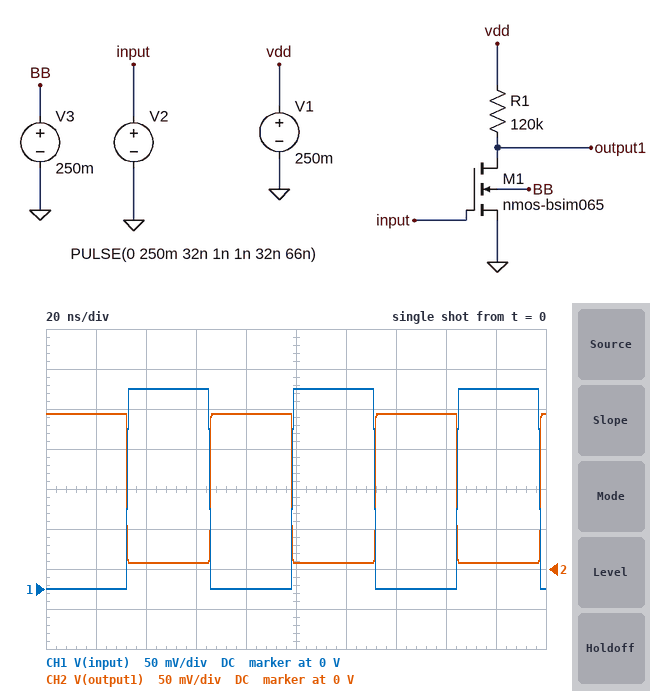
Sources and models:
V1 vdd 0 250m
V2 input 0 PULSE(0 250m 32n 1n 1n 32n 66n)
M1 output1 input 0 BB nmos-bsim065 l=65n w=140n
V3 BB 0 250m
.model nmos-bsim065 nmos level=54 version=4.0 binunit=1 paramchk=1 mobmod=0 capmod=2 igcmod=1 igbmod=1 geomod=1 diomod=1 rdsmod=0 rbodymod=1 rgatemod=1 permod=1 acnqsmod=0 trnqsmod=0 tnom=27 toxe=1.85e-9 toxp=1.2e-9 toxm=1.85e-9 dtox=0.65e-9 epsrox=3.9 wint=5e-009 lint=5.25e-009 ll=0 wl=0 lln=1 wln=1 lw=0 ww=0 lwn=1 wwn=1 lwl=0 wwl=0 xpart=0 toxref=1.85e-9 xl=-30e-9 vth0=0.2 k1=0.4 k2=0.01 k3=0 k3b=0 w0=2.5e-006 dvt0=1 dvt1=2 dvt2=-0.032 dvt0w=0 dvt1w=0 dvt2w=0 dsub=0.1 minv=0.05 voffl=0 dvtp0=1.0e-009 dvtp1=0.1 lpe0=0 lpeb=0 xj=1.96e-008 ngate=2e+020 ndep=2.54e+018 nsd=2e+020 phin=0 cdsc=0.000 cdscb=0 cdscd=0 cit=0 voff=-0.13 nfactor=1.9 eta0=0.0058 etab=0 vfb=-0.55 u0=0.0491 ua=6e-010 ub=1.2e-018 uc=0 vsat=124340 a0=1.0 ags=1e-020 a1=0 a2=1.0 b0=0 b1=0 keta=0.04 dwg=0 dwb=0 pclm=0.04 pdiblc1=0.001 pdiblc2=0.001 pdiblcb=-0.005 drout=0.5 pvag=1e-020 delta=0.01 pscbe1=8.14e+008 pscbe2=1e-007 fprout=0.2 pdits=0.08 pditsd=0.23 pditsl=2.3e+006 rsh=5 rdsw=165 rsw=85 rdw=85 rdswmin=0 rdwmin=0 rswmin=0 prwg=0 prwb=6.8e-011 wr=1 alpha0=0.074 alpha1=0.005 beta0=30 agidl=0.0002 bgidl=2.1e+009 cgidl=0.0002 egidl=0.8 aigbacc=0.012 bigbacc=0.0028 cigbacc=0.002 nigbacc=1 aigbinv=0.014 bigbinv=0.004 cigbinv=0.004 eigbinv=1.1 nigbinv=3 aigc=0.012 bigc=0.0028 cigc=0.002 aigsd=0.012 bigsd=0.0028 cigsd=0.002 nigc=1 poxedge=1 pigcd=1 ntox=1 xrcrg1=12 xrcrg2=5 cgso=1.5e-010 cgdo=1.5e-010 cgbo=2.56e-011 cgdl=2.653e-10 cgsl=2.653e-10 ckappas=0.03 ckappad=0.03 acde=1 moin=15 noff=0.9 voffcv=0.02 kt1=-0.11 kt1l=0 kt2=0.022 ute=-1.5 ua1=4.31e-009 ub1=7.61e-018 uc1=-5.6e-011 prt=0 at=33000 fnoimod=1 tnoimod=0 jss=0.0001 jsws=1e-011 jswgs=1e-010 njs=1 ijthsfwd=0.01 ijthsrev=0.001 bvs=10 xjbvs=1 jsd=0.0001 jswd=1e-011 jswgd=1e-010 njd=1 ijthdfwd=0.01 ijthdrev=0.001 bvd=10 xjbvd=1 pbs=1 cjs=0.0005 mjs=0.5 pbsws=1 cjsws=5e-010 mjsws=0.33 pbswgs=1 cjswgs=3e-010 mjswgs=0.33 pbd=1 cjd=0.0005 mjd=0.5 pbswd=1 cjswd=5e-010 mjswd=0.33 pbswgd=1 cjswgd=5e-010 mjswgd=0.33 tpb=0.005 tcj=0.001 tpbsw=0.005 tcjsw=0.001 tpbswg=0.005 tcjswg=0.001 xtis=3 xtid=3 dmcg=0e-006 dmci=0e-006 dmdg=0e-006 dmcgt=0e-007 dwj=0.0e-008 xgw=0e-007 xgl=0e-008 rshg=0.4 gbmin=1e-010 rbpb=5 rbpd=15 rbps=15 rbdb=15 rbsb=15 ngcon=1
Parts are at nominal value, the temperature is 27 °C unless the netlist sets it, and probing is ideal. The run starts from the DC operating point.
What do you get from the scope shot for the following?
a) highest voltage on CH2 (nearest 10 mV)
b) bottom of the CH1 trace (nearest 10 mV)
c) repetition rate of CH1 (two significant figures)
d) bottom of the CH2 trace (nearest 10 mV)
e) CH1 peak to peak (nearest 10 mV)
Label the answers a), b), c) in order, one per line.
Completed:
a) 190 mV
b) 0 V
c) 15 MHz
d) 10 mV
e) 250 mV
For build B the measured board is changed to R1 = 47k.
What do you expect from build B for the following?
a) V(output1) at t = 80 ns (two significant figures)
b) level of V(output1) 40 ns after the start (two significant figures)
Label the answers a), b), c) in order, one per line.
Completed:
a) 230 mV
b) 19 mV
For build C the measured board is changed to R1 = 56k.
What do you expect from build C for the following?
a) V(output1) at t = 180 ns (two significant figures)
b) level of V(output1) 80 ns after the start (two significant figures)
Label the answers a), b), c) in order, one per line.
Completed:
a) 16 mV
b) 220 mV
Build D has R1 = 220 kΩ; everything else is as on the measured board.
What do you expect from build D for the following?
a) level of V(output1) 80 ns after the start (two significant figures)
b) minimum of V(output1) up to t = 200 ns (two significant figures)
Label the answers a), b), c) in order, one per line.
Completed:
a) 160 mV
b) 3.9 mV
